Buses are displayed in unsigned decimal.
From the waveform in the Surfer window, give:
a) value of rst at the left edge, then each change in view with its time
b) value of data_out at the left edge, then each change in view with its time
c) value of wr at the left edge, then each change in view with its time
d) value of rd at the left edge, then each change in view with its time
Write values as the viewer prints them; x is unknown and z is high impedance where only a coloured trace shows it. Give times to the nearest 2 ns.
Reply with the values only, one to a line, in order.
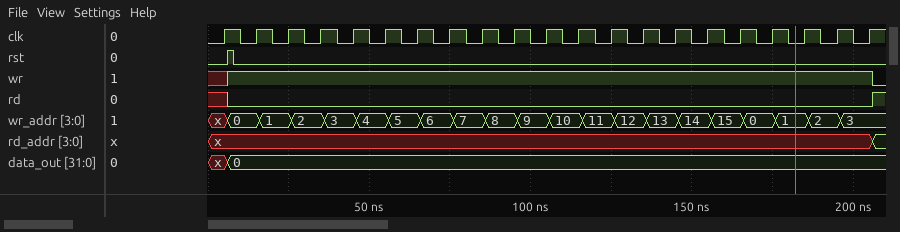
0, 1 at 6 ns, 0 at 8 ns
x, 0 at 6 ns
x, 1 at 6 ns, 0 at 206 ns
x, 0 at 6 ns, 1 at 206 ns
